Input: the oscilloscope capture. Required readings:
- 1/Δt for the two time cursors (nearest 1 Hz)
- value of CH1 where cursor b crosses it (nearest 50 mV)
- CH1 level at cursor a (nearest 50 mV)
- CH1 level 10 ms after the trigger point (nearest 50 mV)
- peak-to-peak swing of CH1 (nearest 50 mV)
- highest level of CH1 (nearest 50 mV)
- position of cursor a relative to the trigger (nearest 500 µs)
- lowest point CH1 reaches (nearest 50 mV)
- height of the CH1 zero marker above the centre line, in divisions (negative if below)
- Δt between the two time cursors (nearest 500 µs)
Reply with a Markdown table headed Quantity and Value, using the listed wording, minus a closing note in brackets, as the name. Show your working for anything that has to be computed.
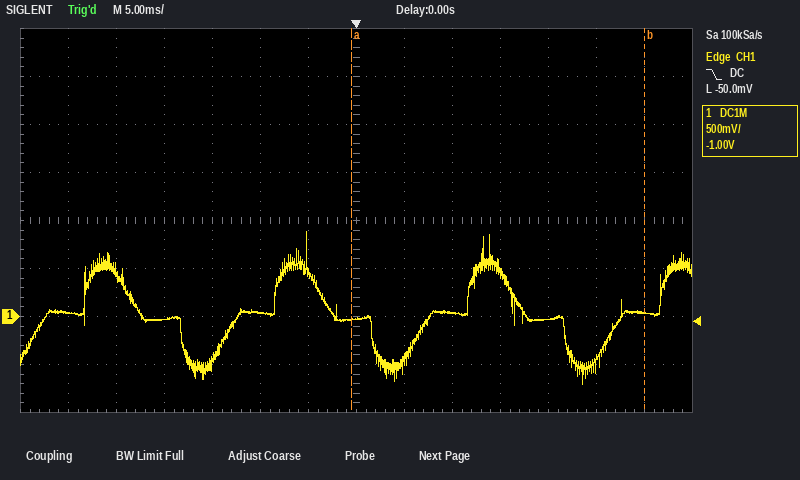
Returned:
| Quantity | Value |
|---|---|
| 1/Δt for the two time cursors | 1 / 30.5 ms ≈ 33 Hz |
| value of CH1 where cursor b crosses it | 50 mV |
| CH1 level at cursor a | -50 mV |
| CH1 level 10 ms after the trigger point | 50 mV |
| peak-to-peak swing of CH1 | 900 mV − (-700 mV) = 1.60 V |
| highest level of CH1 | 900 mV |
| position of cursor a relative to the trigger | -500 µs |
| lowest point CH1 reaches | -700 mV |
| height of the CH1 zero marker above the centre line, in divisions | -2.0 div |
| Δt between the two time cursors | 30.5 ms |
